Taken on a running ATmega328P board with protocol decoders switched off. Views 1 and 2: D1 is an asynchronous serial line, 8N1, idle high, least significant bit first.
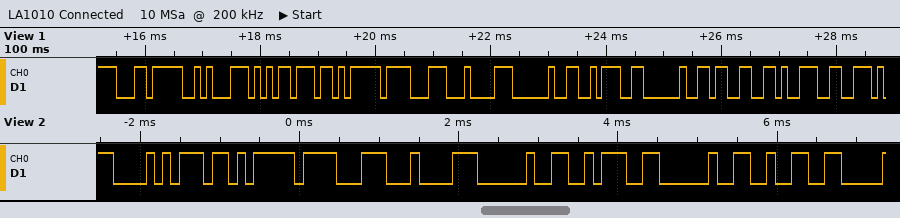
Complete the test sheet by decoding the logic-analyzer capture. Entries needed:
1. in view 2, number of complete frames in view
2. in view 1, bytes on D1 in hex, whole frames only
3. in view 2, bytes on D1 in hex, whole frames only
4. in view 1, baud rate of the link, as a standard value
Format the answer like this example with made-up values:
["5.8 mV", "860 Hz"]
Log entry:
["8", "EC 8A B5 EB 8F 84 20 3A 20 33 39", "A8 EB 8F 84 20 3A 20 32", "9600 baud"]
